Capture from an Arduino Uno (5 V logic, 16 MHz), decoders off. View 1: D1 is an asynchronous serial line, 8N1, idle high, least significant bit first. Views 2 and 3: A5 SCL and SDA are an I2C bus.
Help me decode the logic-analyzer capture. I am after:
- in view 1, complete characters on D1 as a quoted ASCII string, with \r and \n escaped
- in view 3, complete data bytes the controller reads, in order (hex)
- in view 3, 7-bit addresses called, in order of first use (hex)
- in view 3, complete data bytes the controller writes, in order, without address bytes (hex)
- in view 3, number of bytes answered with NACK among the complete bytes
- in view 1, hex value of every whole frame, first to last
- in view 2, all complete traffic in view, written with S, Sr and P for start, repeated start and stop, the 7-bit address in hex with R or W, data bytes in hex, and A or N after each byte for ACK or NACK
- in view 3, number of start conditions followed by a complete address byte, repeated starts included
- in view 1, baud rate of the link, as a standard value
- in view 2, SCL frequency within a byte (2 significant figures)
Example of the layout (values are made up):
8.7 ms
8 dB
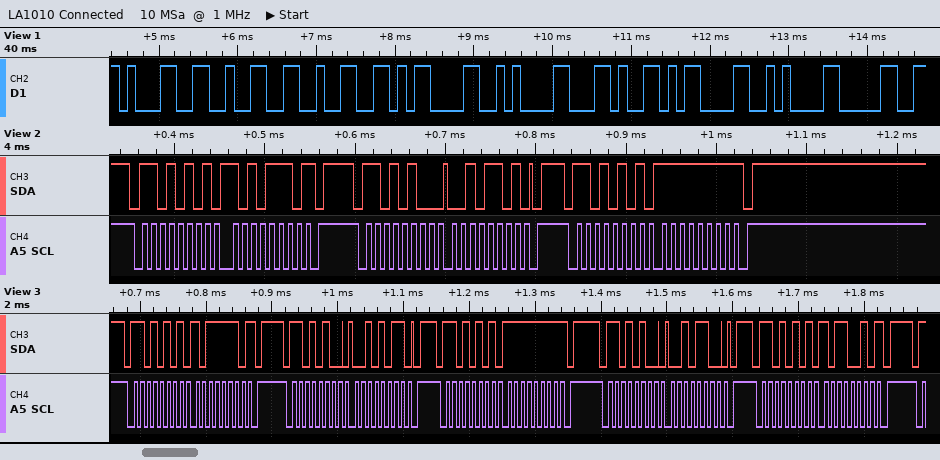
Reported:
"122\r\n,\r\n0"
BE FF B2
0x6A
2B 2C
3
31 32 32 0D 0A 2C 0D 0A 30
S 6AR A AE N P S 6AW A 2D A P S 6AR A FF N P
5
9600 baud
100 kHz
